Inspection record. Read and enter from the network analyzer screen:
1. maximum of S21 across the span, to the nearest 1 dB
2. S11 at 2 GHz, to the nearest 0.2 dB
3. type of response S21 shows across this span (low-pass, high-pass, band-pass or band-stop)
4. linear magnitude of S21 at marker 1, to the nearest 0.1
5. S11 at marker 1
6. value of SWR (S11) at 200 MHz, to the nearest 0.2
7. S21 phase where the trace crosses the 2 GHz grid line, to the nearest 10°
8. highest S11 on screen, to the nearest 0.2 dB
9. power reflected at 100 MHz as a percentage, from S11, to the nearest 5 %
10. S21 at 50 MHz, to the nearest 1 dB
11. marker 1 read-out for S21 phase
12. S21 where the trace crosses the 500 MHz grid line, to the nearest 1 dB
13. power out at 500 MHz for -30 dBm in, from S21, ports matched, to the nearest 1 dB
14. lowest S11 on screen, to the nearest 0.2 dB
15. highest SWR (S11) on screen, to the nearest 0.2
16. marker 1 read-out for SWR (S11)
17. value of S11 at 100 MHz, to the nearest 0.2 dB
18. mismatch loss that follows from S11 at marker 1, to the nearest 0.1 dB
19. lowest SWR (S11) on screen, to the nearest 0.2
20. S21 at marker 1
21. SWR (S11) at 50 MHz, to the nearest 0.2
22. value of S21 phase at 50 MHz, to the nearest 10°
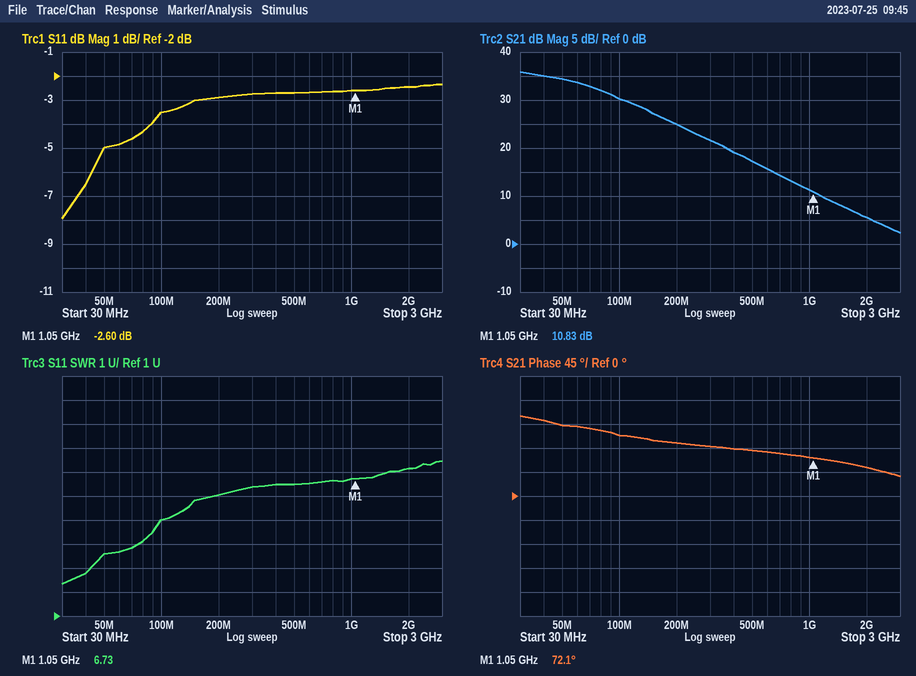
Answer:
36 dB
-2.4 dB
low-pass
3.5
-2.60 dB
6.0
50°
-2.4 dB
45 %
34 dB
72.1°
17 dB
-13 dBm
-8.0 dB
7.4
6.73
-3.6 dB
3.5 dB
2.4
10.83 dB
3.6
130°
